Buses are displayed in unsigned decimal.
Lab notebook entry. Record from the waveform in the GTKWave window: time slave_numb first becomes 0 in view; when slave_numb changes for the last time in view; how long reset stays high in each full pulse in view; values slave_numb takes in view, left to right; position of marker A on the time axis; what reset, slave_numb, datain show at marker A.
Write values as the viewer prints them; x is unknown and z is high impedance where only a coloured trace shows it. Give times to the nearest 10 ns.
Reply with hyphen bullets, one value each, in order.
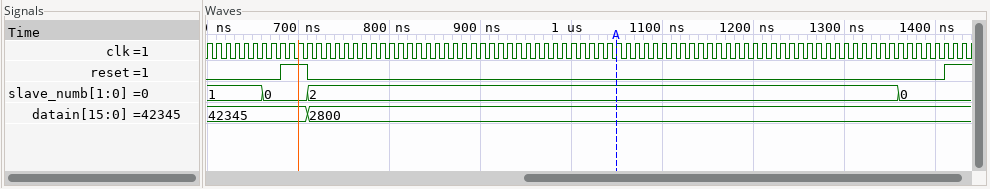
- 660 ns
- 1360 ns
- 30 ns
- 1, 0, 2, 0
- 1050 ns
- reset=0, slave_numb=2, datain=2800
